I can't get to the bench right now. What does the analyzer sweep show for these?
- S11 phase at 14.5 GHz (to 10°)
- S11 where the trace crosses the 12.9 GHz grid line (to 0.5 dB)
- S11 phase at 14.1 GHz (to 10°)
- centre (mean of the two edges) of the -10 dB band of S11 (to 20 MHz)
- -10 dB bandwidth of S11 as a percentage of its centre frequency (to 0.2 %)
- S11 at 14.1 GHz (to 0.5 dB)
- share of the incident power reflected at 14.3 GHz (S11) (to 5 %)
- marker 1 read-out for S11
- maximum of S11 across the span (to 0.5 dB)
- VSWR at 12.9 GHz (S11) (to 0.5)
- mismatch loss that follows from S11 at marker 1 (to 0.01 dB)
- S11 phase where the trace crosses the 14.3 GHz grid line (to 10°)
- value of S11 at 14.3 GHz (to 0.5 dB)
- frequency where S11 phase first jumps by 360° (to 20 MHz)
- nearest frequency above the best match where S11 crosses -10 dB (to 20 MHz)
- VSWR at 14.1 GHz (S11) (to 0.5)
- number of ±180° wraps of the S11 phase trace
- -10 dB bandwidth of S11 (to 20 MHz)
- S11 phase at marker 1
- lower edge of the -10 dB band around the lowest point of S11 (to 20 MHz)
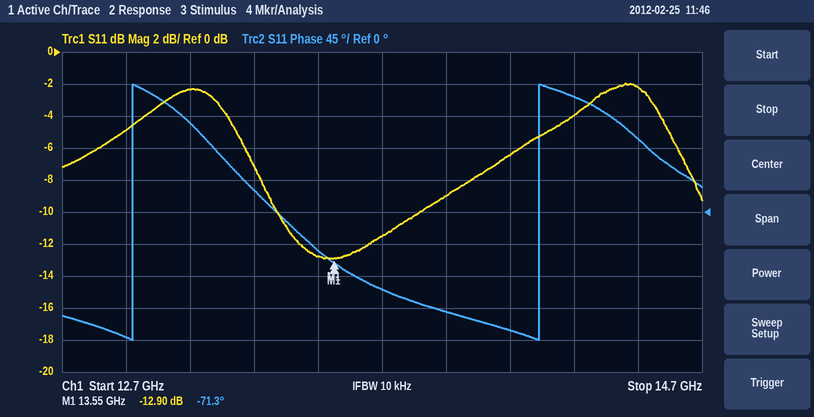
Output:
100°
-5.0 dB
-170°
13.60 GHz
3.2 %
-6.5 dB
40 %
-12.90 dB
-2.0 dB
3.5
0.23 dB
160°
-4.0 dB
12.92 GHz
13.82 GHz
3.0
2
440 MHz
-71.3°
13.38 GHz
